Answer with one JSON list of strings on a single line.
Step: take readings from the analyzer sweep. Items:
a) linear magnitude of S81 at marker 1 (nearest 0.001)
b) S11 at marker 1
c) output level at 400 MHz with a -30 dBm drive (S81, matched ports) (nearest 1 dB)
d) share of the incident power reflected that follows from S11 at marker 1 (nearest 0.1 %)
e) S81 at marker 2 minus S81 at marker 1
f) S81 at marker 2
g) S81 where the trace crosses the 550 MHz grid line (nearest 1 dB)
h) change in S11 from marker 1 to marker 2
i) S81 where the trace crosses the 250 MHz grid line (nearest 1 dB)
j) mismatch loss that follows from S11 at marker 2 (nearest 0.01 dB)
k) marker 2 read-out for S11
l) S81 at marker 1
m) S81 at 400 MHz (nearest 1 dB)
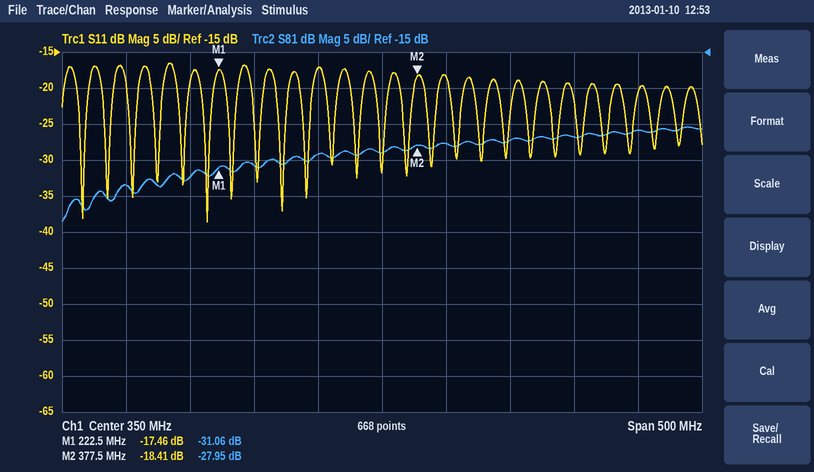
["0.028", "-17.46 dB", "-58 dBm", "1.8 %", "3.11 dB", "-27.95 dB", "-26 dB", "-0.95 dB", "-31 dB", "0.06 dB", "-18.41 dB", "-31.06 dB", "-28 dB"]
